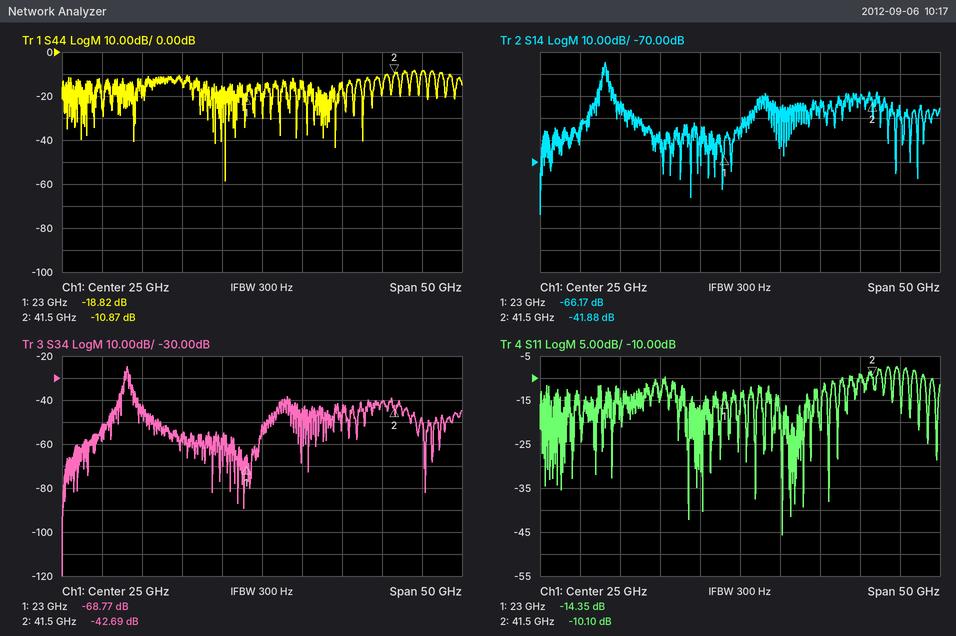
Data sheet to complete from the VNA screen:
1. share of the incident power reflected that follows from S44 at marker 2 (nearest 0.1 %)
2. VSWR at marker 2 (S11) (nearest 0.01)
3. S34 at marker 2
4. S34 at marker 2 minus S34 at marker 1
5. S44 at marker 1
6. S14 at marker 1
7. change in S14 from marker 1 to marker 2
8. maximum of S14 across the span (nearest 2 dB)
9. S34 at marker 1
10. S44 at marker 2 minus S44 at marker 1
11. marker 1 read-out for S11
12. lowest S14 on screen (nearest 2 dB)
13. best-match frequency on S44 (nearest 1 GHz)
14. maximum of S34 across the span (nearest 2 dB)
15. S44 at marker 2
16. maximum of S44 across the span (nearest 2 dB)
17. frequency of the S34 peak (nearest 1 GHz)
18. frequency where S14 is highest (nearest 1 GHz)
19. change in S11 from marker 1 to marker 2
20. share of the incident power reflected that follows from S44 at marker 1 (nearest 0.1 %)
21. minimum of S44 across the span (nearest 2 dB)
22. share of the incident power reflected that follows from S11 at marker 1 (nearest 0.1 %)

8.2 %
1.91
-42.69 dB
26.08 dB
-18.82 dB
-66.17 dB
24.29 dB
-24 dB
-68.77 dB
7.95 dB
-14.35 dB
-94 dB
20 GHz
-24 dB
-10.87 dB
-8 dB
8 GHz
8 GHz
4.25 dB
1.3 %
-58 dB
3.7 %
